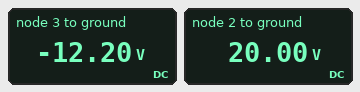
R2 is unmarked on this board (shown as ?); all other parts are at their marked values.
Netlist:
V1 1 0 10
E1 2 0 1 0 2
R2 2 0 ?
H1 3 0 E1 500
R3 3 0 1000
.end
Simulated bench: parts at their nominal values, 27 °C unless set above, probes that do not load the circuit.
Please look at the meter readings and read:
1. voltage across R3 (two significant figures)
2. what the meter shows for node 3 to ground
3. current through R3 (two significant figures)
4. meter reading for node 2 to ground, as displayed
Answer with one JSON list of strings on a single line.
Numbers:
["12 V", "-12.20 V", "12 mA", "20.00 V"]
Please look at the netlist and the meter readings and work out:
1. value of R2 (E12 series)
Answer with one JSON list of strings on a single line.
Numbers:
["820 Ω"]
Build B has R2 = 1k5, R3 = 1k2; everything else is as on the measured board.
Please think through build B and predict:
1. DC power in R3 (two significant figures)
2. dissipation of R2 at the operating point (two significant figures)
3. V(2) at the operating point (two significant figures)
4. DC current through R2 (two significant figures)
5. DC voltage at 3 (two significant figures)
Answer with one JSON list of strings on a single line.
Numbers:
["37 mW", "270 mW", "20 V", "13 mA", "-6.7 V"]
